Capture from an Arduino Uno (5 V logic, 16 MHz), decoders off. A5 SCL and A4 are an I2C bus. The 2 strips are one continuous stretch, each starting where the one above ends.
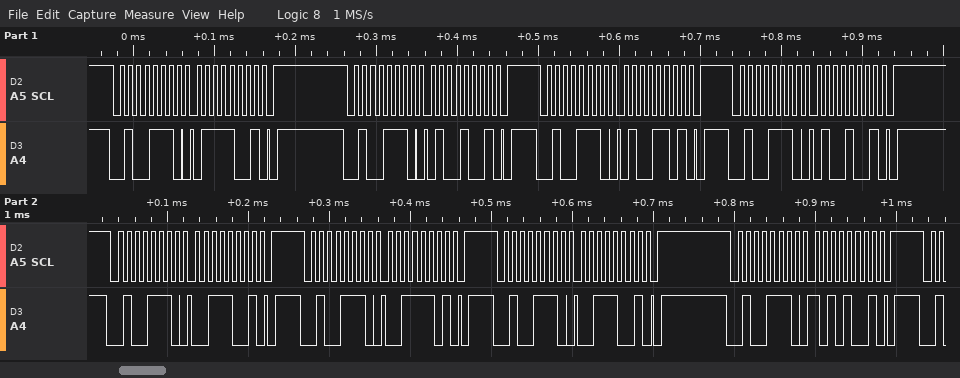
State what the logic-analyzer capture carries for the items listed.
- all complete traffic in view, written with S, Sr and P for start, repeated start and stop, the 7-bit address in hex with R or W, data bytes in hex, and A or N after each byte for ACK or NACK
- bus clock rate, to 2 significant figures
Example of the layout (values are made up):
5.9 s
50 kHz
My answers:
S 27W A 79 A P S 27W A 49 A P S 27W A 4D A P S 27W A 49 A P S 27W A 39 A P S 27W A 3D A P S 27W A 39 A P S 27W A A9 A P
100 kHz
